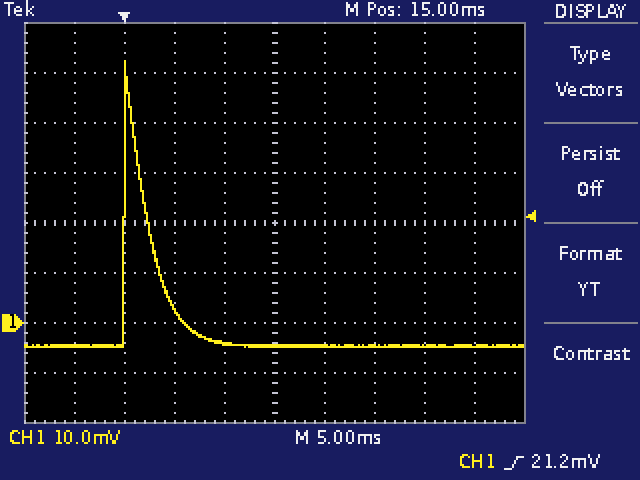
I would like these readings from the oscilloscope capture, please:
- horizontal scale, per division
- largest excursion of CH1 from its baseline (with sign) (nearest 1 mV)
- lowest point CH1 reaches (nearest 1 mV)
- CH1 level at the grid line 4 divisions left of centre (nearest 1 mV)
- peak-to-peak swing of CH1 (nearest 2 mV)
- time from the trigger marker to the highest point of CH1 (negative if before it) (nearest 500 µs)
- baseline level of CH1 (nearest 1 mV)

5 ms
+57 mV
-5 mV
-5 mV
58 mV
0.0 ms
-5 mV
